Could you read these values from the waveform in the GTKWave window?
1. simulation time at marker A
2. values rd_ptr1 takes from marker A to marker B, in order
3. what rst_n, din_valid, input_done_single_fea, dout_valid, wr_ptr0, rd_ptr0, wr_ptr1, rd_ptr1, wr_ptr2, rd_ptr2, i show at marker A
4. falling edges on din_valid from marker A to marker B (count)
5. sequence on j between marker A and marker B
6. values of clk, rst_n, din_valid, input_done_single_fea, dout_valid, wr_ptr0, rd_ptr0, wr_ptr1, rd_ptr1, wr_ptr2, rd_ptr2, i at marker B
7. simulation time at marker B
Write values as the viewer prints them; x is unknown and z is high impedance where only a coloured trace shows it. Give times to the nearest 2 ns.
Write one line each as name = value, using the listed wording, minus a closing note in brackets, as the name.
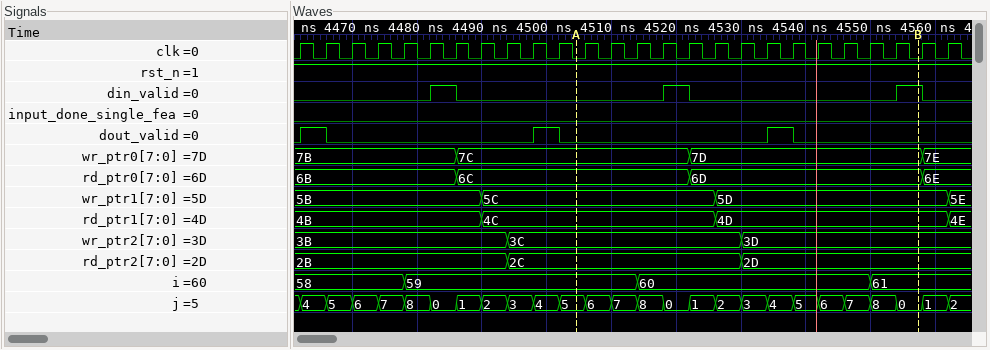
simulation time at marker A = 4504 ns
values rd_ptr1 takes from marker A to marker B, in order = 4C, 4D
what rst_n, din_valid, input_done_single_fea, dout_valid, wr_ptr0, rd_ptr0, wr_ptr1, rd_ptr1, wr_ptr2, rd_ptr2, i show at marker A = rst_n=1, din_valid=0, input_done_single_fea=0, dout_valid=0, wr_ptr0=7C, rd_ptr0=6C, wr_ptr1=5C, rd_ptr1=4C, wr_ptr2=3C, rd_ptr2=2C, i=59
falling edges on din_valid from marker A to marker B = 1
sequence on j between marker A and marker B = 5, 6, 7, 8, 0, 1, 2, 3, 4, 5, 6, 7, 8, 0
values of clk, rst_n, din_valid, input_done_single_fea, dout_valid, wr_ptr0, rd_ptr0, wr_ptr1, rd_ptr1, wr_ptr2, rd_ptr2, i at marker B = clk=0, rst_n=1, din_valid=1, input_done_single_fea=0, dout_valid=0, wr_ptr0=7D, rd_ptr0=6D, wr_ptr1=5D, rd_ptr1=4D, wr_ptr2=3D, rd_ptr2=2D, i=61
simulation time at marker B = 4558 ns
